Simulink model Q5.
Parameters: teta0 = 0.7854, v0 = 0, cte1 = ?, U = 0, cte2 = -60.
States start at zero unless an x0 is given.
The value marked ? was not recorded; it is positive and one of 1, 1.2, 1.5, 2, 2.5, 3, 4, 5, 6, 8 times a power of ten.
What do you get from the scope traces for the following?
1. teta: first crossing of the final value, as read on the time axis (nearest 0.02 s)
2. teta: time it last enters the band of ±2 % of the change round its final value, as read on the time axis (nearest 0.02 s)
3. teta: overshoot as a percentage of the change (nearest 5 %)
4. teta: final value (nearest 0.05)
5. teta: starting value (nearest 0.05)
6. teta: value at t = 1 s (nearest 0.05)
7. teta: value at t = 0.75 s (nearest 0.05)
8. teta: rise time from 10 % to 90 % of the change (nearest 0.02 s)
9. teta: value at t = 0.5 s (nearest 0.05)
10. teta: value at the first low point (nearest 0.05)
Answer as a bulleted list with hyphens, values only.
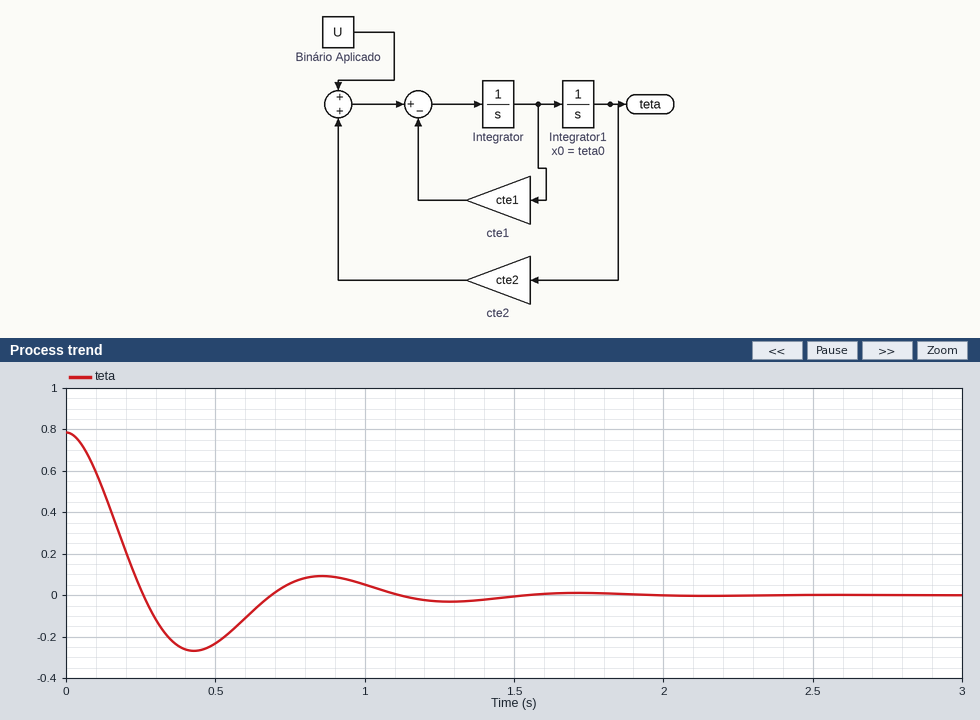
- 0.26 s
- 1.44 s
- 35 %
- 0.00
- 0.80
- 0.05
- 0.05
- 0.18 s
- -0.25
- -0.25
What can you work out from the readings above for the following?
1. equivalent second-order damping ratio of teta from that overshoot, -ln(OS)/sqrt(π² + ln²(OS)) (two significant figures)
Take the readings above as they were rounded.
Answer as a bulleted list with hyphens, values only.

- 0.32
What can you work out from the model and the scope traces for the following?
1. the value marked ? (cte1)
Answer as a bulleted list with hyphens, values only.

- 5
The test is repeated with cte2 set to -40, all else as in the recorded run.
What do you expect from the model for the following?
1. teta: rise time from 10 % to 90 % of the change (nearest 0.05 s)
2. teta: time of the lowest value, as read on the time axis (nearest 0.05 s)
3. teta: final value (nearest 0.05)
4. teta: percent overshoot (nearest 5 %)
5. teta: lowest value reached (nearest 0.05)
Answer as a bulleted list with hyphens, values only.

- 0.25 s
- 0.55 s
- 0.00
- 25 %
- -0.20
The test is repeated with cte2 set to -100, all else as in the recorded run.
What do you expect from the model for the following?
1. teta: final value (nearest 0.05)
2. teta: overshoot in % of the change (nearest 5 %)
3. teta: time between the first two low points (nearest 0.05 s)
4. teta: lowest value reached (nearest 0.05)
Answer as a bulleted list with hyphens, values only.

- 0.00
- 45 %
- 0.65 s
- -0.35
